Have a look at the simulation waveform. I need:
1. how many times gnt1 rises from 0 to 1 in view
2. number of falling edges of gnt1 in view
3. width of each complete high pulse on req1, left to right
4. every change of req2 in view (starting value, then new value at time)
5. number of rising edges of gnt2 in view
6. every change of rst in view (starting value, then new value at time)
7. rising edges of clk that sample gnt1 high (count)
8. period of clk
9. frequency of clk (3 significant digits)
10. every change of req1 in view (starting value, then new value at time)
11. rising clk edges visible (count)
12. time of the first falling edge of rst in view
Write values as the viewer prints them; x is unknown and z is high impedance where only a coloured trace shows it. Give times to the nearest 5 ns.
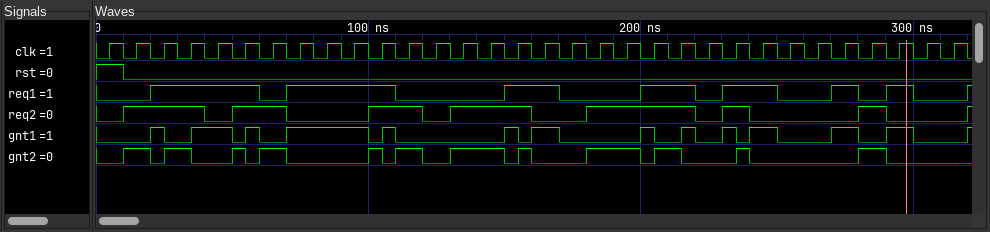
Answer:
14
13
40 ns, 40 ns, 20 ns, 20 ns, 20 ns, 10 ns, 10 ns
0, 1 at 10 ns, 0 at 40 ns, 1 at 50 ns, 0 at 70 ns, 1 at 100 ns, 0 at 120 ns, 1 at 130 ns, 0 at 160 ns, 1 at 180 ns, 0 at 220 ns, 1 at 230 ns, 0 at 240 ns, 1 at 280 ns, 0 at 290 ns, 1 at 320 ns
12
1, 0 at 10 ns
12
10 ns
100 MHz
0, 1 at 20 ns, 0 at 60 ns, 1 at 70 ns, 0 at 110 ns, 1 at 150 ns, 0 at 170 ns, 1 at 200 ns, 0 at 220 ns, 1 at 230 ns, 0 at 250 ns, 1 at 270 ns, 0 at 280 ns, 1 at 290 ns, 0 at 300 ns, 1 at 320 ns
32
10 ns
